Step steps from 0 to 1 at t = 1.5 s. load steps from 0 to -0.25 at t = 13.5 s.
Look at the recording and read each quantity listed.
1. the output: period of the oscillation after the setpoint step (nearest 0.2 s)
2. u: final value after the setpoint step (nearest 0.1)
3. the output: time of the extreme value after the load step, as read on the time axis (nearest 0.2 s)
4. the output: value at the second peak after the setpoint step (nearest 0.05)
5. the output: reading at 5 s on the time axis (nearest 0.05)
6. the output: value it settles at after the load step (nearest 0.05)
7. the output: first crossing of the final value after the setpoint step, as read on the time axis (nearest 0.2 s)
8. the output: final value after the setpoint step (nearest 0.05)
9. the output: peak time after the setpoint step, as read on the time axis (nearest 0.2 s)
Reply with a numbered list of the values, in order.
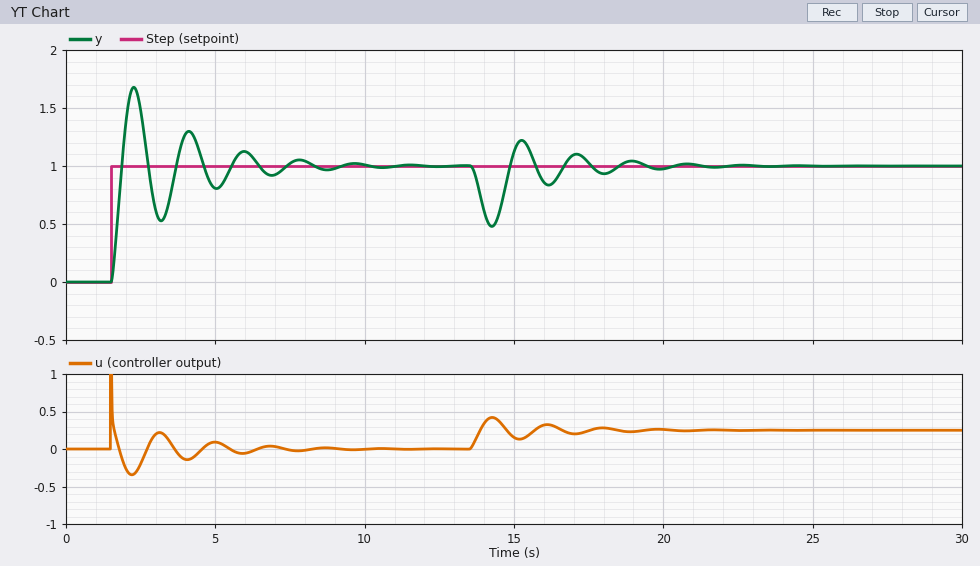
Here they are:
1. 1.8 s
2. 0.0
3. 14.2 s
4. 1.30
5. 0.80
6. 1.00
7. 1.8 s
8. 1.00
9. 2.2 s
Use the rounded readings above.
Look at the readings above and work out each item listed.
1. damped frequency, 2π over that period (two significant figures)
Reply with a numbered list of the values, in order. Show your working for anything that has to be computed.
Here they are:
1. 2π / 1.8 = 3.5 rad/s
